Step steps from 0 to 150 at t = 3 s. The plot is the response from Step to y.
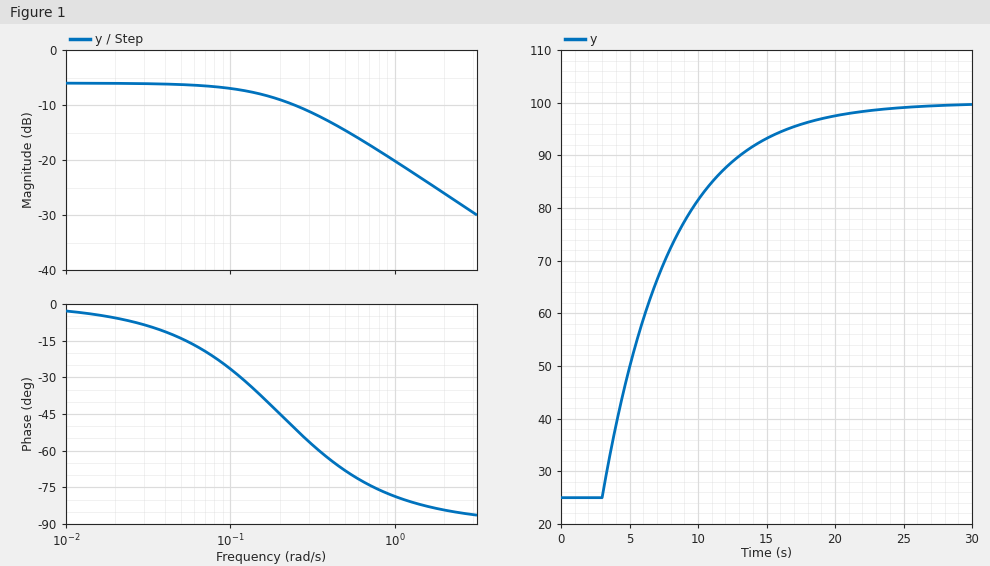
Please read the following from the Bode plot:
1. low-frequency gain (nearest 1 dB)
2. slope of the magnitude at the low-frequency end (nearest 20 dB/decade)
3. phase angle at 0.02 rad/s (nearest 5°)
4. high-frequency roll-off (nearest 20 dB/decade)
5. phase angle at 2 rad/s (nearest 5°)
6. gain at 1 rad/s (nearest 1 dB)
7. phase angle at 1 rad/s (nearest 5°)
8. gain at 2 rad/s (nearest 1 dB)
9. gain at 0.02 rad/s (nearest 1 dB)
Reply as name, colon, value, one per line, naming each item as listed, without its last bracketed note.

low-frequency gain: -6 dB
slope of the magnitude at the low-frequency end: 0 dB/decade
phase angle at 0.02 rad/s: -5°
high-frequency roll-off: -20 dB/decade
phase angle at 2 rad/s: -85°
gain at 1 rad/s: -20 dB
phase angle at 1 rad/s: -80°
gain at 2 rad/s: -26 dB
gain at 0.02 rad/s: -6 dB
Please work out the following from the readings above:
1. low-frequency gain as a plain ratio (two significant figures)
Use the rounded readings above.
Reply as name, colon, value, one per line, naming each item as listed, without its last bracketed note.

low-frequency gain as a plain ratio: 0.50
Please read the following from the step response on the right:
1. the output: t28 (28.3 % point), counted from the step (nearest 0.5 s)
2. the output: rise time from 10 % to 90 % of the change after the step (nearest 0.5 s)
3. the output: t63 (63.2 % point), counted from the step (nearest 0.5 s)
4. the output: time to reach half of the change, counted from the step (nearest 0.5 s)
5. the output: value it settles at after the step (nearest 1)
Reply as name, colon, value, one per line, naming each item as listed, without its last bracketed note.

the output: t28 (28.3 % point), counted from the step: 1.5 s
the output: rise time from 10 % to 90 % of the change after the step: 11.0 s
the output: t63 (63.2 % point), counted from the step: 5.0 s
the output: time to reach half of the change, counted from the step: 3.5 s
the output: value it settles at after the step: 100
